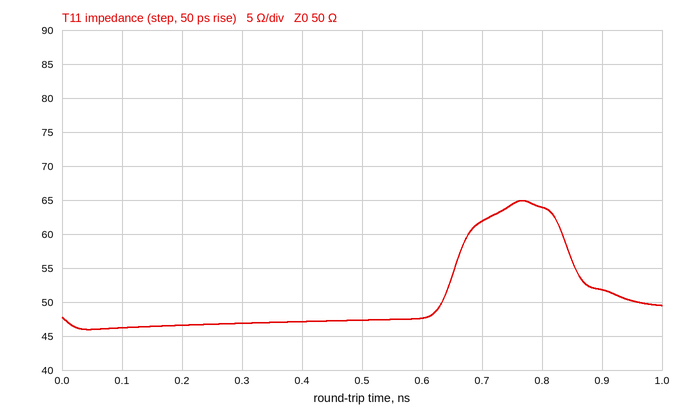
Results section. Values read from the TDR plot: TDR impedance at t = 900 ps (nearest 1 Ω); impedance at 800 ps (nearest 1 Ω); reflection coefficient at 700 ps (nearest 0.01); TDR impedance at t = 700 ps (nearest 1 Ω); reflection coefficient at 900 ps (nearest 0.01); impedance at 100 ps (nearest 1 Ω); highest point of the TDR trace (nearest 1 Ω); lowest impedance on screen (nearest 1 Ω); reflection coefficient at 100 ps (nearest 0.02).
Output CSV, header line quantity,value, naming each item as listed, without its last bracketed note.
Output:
quantity,value
TDR impedance at t = 900 ps,52 Ω
impedance at 800 ps,64 Ω
reflection coefficient at 700 ps,+0.11
TDR impedance at t = 700 ps,62 Ω
reflection coefficient at 900 ps,+0.02
impedance at 100 ps,46 Ω
highest point of the TDR trace,65 Ω
lowest impedance on screen,46 Ω
reflection coefficient at 100 ps,-0.04
